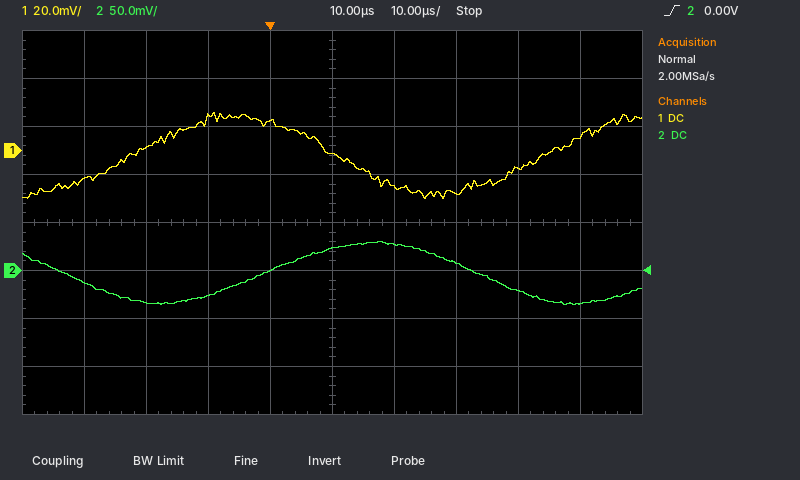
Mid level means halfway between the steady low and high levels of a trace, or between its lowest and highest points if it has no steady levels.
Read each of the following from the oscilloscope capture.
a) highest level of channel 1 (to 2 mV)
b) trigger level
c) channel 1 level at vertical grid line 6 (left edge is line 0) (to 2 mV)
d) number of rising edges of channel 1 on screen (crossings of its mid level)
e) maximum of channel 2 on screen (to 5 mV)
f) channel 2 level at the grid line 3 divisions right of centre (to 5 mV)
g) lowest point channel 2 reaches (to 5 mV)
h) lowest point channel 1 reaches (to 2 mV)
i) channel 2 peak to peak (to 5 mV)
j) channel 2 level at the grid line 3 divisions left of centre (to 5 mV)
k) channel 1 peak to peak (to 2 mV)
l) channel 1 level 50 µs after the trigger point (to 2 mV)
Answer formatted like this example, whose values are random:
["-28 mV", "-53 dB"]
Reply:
["16 mV", "0.00 V", "-16 mV", "2", "30 mV", "-20 mV", "-35 mV", "-20 mV", "65 mV", "-35 mV", "36 mV", "6 mV"]
